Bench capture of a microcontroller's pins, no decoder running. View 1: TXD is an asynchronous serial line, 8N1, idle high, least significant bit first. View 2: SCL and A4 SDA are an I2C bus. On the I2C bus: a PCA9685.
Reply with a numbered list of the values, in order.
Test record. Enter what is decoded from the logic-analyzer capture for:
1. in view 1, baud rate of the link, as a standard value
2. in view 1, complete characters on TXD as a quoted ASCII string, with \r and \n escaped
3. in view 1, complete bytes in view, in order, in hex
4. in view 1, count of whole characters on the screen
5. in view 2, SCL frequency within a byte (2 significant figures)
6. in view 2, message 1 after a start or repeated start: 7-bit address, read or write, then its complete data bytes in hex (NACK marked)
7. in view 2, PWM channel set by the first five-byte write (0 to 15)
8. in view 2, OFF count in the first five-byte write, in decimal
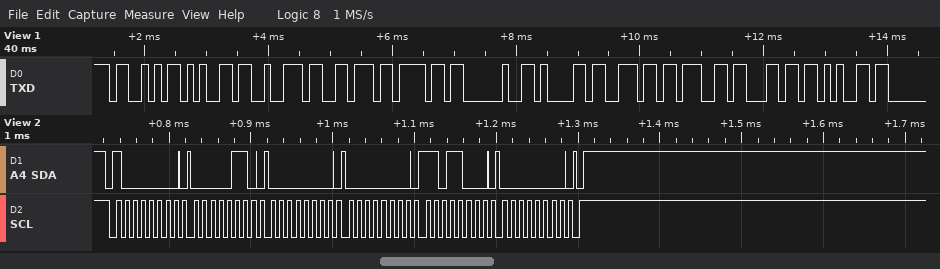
1. 9600 baud
2. "Servo angle"
3. 53 65 72 76 6F 20 61 6E 67 6C 65
4. 11
5. 100 kHz
6. 0x40 write: 06 00 00 D8 00
7. 0
8. 216
